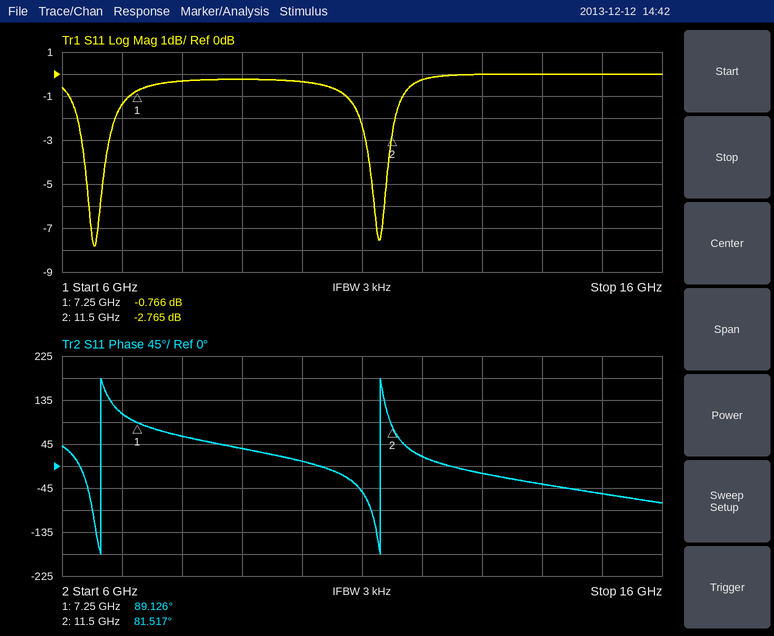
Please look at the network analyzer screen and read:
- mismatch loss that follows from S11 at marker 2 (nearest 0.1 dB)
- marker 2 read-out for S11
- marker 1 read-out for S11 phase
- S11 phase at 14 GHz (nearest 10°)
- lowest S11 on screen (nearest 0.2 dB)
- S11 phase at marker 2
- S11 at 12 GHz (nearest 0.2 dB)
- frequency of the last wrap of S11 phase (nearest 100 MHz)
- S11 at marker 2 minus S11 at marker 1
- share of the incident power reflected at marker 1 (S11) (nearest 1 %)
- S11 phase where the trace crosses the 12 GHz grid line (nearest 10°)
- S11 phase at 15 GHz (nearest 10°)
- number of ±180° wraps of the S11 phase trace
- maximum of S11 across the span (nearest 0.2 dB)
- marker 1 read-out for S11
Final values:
3.3 dB
-2.765 dB
89.126°
-40°
-7.8 dB
81.517°
-0.2 dB
11.3 GHz
-1.999 dB
84 %
20°
-60°
2
0.0 dB
-0.766 dB
